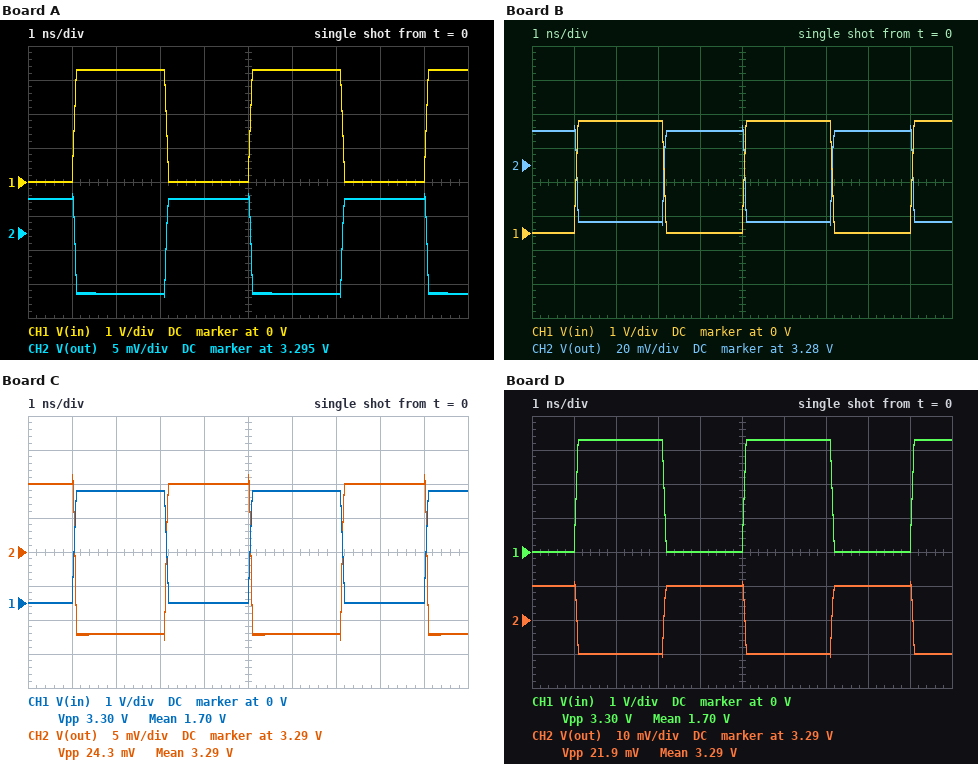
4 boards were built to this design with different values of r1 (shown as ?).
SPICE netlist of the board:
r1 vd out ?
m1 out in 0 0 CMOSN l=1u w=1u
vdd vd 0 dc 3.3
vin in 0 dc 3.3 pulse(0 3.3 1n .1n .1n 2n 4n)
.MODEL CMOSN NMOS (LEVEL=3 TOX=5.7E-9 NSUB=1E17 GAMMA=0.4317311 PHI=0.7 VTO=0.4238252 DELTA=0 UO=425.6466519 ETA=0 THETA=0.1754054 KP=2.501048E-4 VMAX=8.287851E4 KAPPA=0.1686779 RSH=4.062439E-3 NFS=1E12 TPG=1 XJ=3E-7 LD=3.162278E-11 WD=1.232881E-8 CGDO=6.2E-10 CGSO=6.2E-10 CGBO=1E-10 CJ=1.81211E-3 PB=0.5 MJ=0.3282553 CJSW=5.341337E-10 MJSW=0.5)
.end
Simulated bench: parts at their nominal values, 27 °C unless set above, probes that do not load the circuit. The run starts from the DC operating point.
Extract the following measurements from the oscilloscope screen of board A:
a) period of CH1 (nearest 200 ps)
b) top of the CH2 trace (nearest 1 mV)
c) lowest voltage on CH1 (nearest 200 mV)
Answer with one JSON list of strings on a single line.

["4.0 ns", "3.301 V", "0 V"]
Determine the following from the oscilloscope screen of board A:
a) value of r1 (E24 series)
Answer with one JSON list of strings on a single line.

["39 Ω"]
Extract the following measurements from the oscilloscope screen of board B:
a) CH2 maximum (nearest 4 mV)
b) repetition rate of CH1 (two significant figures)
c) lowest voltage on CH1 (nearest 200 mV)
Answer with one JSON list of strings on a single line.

["3.304 V", "250 MHz", "0 V"]
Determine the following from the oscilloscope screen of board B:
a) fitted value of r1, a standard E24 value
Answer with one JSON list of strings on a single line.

["150 Ω"]
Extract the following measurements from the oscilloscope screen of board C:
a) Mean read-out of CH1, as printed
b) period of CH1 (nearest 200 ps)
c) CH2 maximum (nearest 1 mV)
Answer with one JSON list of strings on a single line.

["1.70 V", "4.0 ns", "3.301 V"]
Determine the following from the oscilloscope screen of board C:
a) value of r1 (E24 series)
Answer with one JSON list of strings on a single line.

["62 Ω"]
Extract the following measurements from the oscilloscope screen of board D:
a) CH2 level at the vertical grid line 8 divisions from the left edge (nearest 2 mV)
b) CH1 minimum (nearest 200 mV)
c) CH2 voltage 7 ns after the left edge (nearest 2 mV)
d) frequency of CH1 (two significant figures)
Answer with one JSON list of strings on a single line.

["3.300 V", "0 V", "3.280 V", "250 MHz"]
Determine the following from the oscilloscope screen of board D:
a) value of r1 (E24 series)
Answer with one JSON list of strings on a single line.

["56 Ω"]
